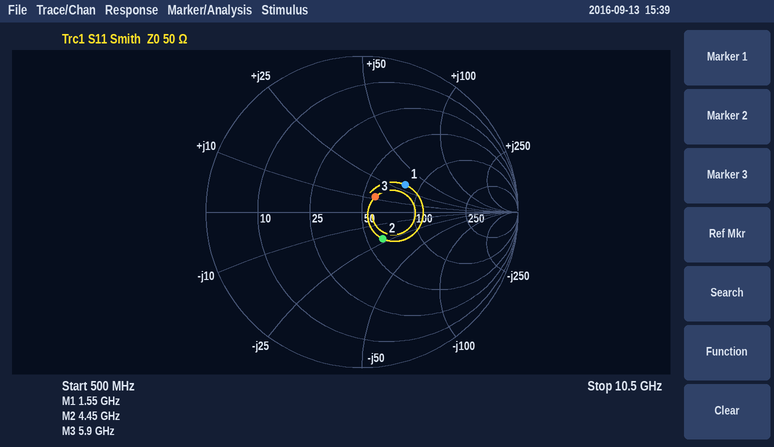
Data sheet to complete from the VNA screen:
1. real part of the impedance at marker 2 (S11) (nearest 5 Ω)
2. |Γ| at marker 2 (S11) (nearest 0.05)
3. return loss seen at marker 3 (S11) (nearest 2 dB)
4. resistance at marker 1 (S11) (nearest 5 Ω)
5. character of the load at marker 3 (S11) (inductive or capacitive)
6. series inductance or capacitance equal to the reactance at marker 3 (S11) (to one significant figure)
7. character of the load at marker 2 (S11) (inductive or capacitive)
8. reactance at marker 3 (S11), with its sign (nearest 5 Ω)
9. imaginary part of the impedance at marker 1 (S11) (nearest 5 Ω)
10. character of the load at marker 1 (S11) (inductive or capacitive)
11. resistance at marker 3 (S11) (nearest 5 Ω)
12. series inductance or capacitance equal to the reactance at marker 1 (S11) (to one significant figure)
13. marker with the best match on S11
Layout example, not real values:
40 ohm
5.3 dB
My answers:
60 Ω
0.20
18 dB
80 Ω
inductive
300 pH
capacitive
+10 Ω
+30 Ω
inductive
60 Ω
3 nH
marker 3
